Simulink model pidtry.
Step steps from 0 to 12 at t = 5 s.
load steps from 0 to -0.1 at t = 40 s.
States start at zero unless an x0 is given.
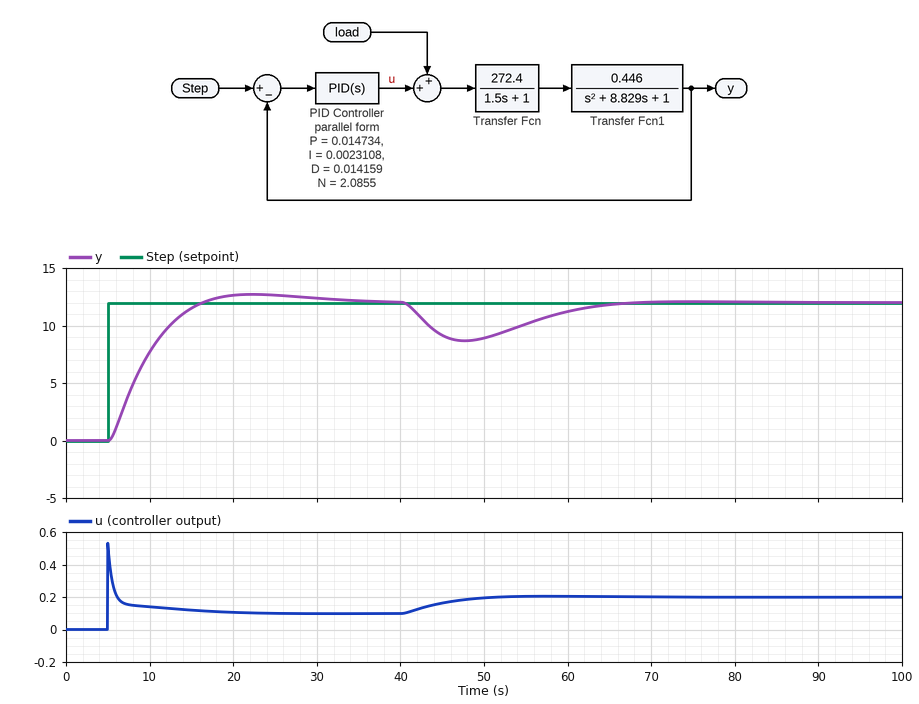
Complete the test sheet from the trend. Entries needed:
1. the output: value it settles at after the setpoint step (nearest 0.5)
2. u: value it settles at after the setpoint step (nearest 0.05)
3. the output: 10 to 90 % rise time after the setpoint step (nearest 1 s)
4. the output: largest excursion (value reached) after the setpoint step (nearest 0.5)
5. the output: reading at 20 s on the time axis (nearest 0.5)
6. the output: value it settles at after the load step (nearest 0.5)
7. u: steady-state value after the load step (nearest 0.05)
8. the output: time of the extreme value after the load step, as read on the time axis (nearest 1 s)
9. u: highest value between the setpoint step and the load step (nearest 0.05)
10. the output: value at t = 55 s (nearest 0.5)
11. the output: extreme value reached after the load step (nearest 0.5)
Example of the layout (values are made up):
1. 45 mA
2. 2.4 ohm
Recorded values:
1. 12.0
2. 0.10
3. 8 s
4. 12.5
5. 12.5
6. 12.0
7. 0.20
8. 48 s
9. 0.55
10. 10.0
11. 8.5
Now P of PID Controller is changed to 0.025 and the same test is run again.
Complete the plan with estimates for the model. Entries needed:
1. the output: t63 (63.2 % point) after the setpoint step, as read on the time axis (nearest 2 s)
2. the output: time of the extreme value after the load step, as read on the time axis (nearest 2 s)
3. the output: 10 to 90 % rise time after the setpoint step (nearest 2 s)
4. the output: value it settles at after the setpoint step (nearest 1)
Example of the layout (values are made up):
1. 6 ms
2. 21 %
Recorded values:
1. 8 s
2. 46 s
3. 6 s
4. 12
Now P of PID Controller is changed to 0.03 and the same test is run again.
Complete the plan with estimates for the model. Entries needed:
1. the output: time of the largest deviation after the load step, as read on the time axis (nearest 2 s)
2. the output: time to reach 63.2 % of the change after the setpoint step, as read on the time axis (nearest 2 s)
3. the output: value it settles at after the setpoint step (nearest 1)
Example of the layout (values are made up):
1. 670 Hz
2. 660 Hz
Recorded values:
1. 46 s
2. 8 s
3. 12
